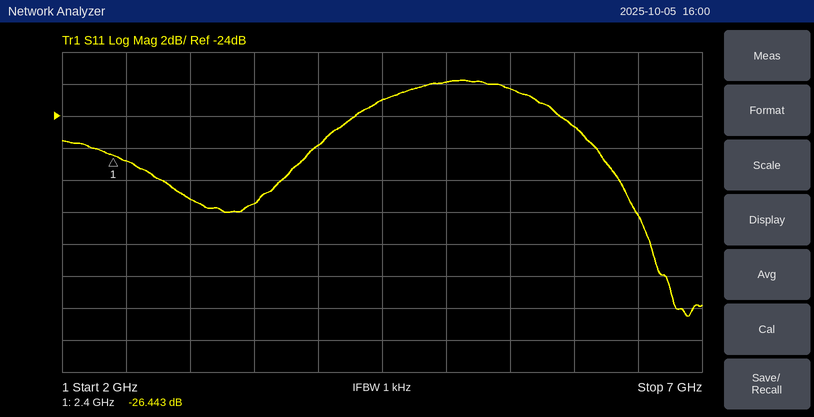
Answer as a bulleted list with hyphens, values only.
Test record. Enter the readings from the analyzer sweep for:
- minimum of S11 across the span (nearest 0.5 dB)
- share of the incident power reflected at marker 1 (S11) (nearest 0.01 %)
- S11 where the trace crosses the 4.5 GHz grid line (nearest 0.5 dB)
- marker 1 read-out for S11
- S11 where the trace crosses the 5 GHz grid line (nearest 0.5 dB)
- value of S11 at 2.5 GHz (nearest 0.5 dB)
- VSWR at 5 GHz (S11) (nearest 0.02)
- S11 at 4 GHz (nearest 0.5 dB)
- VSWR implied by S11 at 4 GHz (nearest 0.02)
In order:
- -36.5 dB
- 0.23 %
- -23.0 dB
- -26.443 dB
- -22.0 dB
- -27.0 dB
- 1.18
- -26.0 dB
- 1.10
